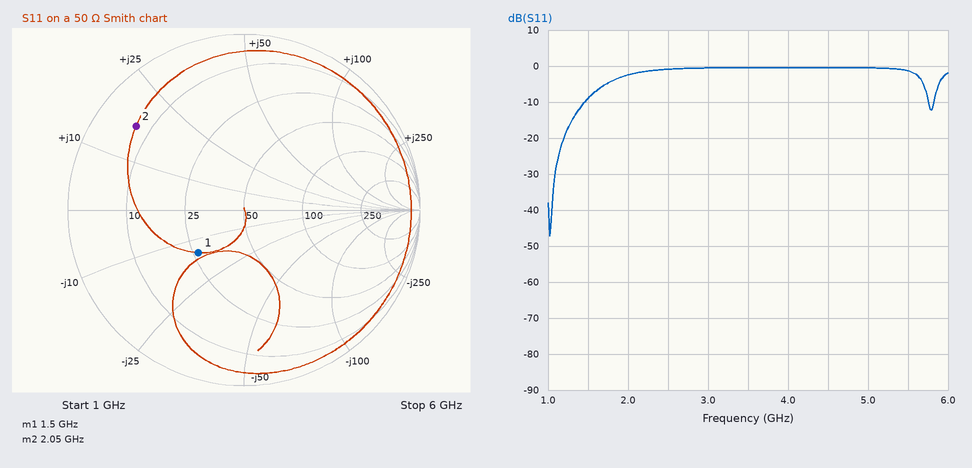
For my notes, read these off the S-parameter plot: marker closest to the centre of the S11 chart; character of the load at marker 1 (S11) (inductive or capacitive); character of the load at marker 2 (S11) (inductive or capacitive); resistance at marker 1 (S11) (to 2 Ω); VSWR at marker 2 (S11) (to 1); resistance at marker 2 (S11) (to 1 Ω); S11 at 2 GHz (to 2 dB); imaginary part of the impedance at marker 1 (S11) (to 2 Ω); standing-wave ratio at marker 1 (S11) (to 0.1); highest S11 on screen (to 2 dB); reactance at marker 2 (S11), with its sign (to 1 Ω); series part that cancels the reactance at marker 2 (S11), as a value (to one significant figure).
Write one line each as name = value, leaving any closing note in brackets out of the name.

marker closest to the centre of the S11 chart = marker 1
character of the load at marker 1 (S11) = capacitive
character of the load at marker 2 (S11) = inductive
resistance at marker 1 (S11) = 26 Ω
VSWR at marker 2 (S11) = 8
resistance at marker 2 (S11) = 7 Ω
S11 at 2 GHz = -2 dB
imaginary part of the impedance at marker 1 (S11) = -14 Ω
standing-wave ratio at marker 1 (S11) = 2.1
highest S11 on screen = 0 dB
reactance at marker 2 (S11), with its sign = +17 Ω
series part that cancels the reactance at marker 2 (S11), as a value = 5 pF
